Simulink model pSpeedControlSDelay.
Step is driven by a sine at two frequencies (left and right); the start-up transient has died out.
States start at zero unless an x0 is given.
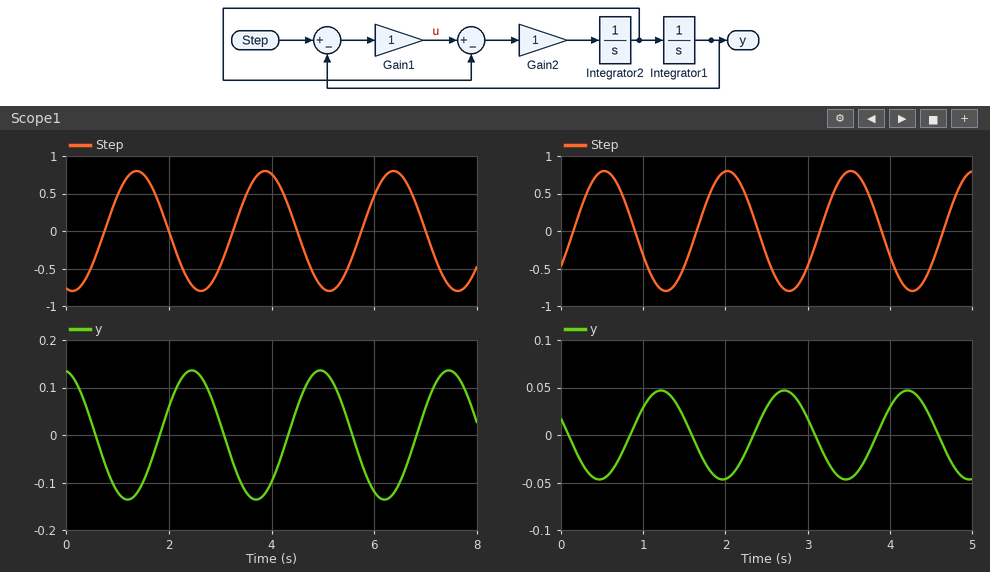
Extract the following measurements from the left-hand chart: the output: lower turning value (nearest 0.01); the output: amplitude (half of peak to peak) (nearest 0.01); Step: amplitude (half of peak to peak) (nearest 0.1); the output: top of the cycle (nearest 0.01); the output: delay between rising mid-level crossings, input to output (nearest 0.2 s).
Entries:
-0.14
0.14
0.8
0.14
1.0 s
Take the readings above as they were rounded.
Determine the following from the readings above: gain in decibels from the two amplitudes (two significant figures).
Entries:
-15 dB
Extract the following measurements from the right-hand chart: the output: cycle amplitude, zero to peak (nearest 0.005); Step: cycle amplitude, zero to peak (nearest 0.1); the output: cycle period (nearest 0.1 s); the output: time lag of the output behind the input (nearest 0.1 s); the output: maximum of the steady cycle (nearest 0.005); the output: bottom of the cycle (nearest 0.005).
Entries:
0.045
0.8
1.5 s
0.7 s
0.045
-0.045
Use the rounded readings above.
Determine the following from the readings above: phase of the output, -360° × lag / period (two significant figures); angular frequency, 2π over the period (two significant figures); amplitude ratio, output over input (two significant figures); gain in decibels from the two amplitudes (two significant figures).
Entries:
-170°
4.2 rad/s
0.056
-25 dB
